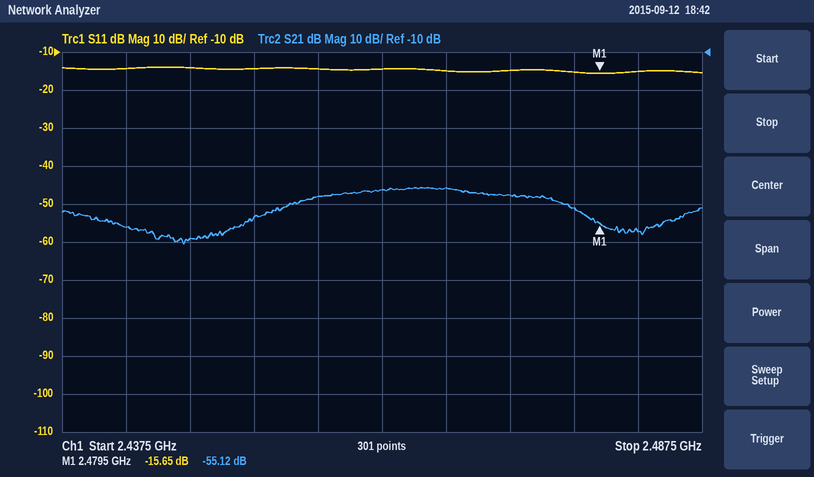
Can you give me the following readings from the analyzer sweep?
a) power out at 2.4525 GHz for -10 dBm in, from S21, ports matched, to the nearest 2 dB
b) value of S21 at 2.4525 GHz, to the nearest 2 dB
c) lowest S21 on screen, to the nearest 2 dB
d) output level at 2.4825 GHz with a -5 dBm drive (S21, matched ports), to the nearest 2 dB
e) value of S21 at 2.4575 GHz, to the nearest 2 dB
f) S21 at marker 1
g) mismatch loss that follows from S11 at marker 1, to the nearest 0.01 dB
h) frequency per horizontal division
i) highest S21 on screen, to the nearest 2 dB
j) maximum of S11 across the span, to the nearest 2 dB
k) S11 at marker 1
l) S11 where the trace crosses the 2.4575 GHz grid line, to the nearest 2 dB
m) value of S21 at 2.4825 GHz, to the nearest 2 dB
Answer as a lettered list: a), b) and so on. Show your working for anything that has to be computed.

a) -10 dBm + (-54 dB) = -64 dBm
b) -54 dB
c) -60 dB
d) -5 dBm + (-58 dB) = -62 dBm
e) -48 dB
f) -55.12 dB
g) −10 log10(1 − 10^(-15.65/10)) ≈ 0.12 dB
h) 5 MHz
i) -46 dB
j) -14 dB
k) -15.65 dB
l) -14 dB
m) -58 dB
